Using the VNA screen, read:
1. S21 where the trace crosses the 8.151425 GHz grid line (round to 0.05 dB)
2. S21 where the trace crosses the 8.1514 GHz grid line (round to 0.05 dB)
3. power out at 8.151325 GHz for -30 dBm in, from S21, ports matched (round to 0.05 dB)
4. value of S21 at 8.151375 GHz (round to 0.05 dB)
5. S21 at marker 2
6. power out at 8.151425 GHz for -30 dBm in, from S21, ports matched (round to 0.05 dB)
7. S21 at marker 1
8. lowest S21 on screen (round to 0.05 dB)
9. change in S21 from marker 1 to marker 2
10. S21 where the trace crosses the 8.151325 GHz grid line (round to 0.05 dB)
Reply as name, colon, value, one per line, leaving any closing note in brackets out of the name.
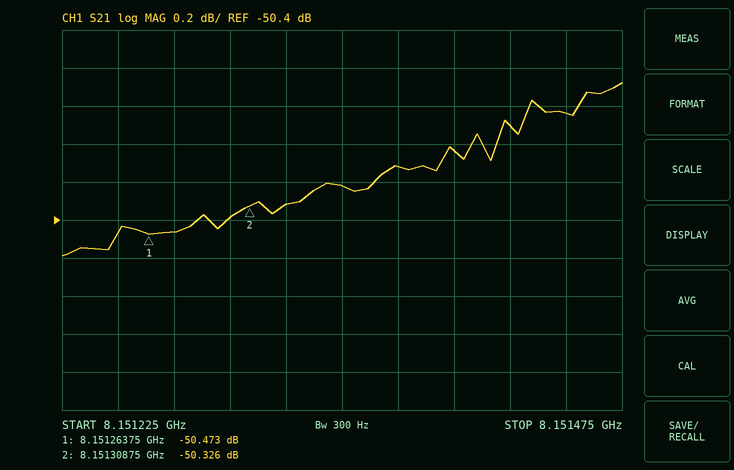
S21 where the trace crosses the 8.151425 GHz grid line: -49.90 dB
S21 where the trace crosses the 8.1514 GHz grid line: -50.05 dB
power out at 8.151325 GHz for -30 dBm in, from S21, ports matched: -80.30 dBm
value of S21 at 8.151375 GHz: -50.10 dB
S21 at marker 2: -50.326 dB
power out at 8.151425 GHz for -30 dBm in, from S21, ports matched: -79.90 dBm
S21 at marker 1: -50.473 dB
lowest S21 on screen: -50.60 dB
change in S21 from marker 1 to marker 2: 0.147 dB
S21 where the trace crosses the 8.151325 GHz grid line: -50.30 dB
